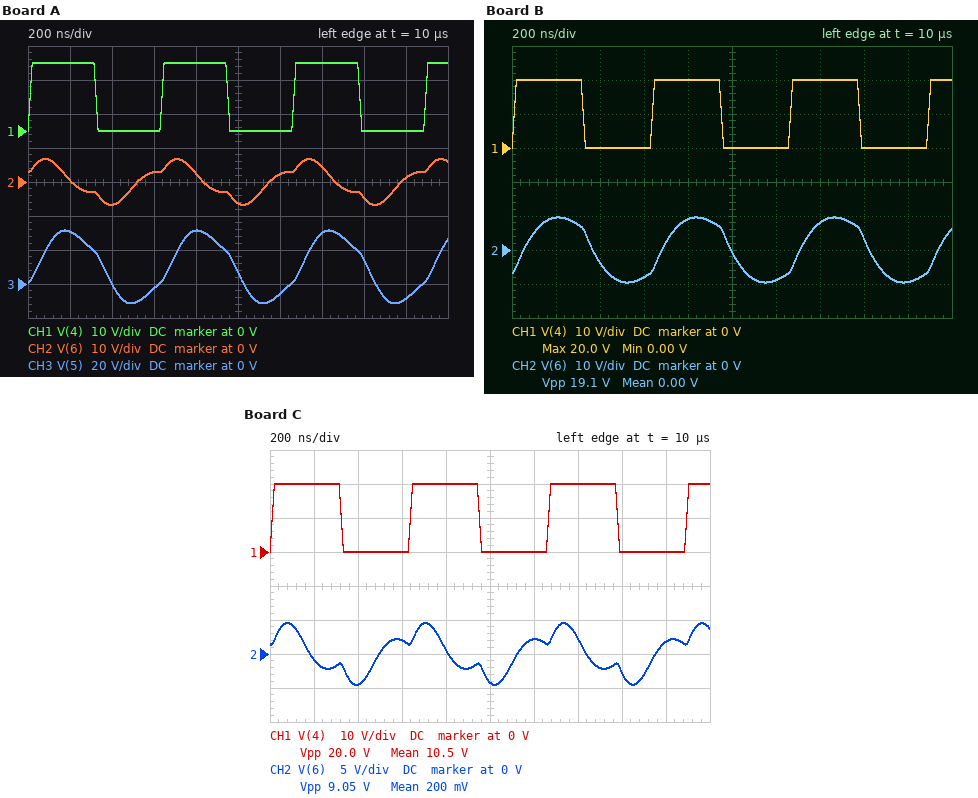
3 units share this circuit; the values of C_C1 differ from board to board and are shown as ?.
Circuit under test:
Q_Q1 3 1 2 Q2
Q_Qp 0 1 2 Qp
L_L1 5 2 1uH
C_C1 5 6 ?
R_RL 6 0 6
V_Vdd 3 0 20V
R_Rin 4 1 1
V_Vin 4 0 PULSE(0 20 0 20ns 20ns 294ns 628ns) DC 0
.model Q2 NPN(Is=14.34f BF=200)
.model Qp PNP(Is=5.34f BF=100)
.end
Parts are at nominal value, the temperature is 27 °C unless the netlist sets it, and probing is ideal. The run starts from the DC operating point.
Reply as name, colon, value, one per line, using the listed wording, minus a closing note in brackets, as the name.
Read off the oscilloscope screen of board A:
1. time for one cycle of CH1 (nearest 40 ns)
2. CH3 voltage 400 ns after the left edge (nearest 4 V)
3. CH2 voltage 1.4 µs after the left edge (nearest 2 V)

time for one cycle of CH1: 640 ns
CH3 voltage 400 ns after the left edge: 0 V
CH2 voltage 1.4 µs after the left edge: 4 V
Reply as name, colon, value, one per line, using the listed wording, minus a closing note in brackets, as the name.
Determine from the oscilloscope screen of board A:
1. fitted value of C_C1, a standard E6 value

fitted value of C_C1, a standard E6 value: 4.7 nF
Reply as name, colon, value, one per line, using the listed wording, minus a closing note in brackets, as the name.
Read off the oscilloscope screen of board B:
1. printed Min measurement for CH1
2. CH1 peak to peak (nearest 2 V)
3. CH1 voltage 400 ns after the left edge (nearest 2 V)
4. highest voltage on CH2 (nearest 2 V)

printed Min measurement for CH1: 0.00 V
CH1 peak to peak: 20 V
CH1 voltage 400 ns after the left edge: 0 V
highest voltage on CH2: 10 V
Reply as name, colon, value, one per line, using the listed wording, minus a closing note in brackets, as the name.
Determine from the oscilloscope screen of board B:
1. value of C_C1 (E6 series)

value of C_C1: 15 nF
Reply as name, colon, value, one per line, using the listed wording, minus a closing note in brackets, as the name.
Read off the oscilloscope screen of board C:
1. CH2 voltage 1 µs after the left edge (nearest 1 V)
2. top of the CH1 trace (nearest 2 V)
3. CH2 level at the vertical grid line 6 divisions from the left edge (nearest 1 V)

CH2 voltage 1 µs after the left edge: -4 V
top of the CH1 trace: 20 V
CH2 level at the vertical grid line 6 divisions from the left edge: 2 V
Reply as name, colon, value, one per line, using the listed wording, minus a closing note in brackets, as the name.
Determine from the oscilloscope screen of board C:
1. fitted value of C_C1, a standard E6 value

fitted value of C_C1, a standard E6 value: 3.3 nF
